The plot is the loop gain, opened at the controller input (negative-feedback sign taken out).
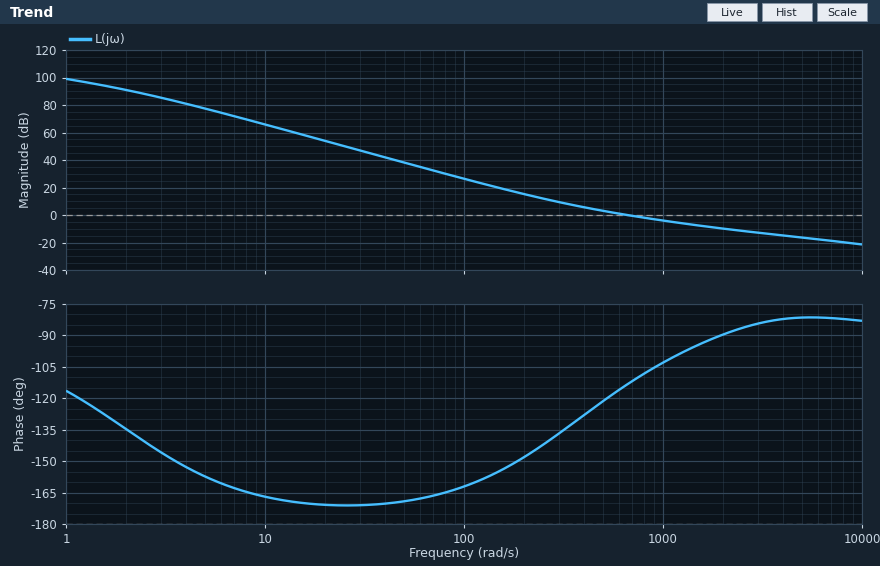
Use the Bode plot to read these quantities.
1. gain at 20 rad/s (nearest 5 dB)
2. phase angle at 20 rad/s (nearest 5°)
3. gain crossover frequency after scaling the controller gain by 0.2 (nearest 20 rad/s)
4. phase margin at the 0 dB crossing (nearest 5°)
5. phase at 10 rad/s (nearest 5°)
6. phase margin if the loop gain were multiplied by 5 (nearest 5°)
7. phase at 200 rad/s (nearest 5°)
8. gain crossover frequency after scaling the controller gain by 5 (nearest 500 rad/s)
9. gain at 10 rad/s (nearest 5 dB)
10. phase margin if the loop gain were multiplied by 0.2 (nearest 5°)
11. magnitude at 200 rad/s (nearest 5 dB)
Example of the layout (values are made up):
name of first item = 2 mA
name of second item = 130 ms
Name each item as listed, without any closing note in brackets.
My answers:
gain at 20 rad/s = 55 dB
phase angle at 20 rad/s = -170°
gain crossover frequency after scaling the controller gain by 0.2 = 220 rad/s
phase margin at the 0 dB crossing = 65°
phase at 10 rad/s = -165°
phase margin if the loop gain were multiplied by 5 = 95°
phase at 200 rad/s = -150°
gain crossover frequency after scaling the controller gain by 5 = 3500 rad/s
gain at 10 rad/s = 65 dB
phase margin if the loop gain were multiplied by 0.2 = 35°
magnitude at 200 rad/s = 15 dB
